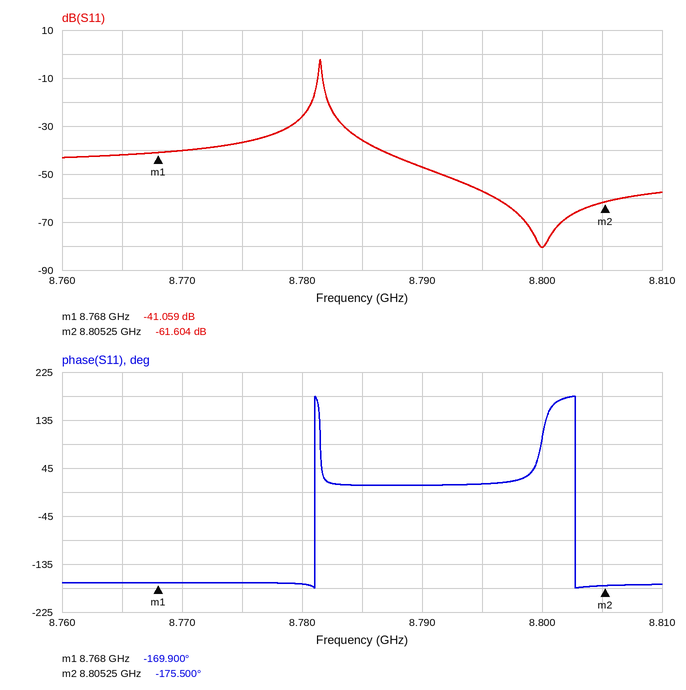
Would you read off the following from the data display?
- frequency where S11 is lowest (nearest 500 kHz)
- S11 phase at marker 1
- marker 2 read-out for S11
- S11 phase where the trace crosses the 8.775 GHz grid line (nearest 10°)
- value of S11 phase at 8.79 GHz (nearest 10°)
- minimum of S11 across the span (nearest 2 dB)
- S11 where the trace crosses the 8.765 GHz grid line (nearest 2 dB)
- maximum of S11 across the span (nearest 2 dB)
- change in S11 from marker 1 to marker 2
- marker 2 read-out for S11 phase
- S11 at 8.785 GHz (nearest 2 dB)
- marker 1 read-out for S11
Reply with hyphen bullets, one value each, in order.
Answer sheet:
- 8.8000 GHz
- -169.900°
- -61.604 dB
- -170°
- 10°
- -80 dB
- -42 dB
- -2 dB
- -20.545 dB
- -175.500°
- -36 dB
- -41.059 dB
